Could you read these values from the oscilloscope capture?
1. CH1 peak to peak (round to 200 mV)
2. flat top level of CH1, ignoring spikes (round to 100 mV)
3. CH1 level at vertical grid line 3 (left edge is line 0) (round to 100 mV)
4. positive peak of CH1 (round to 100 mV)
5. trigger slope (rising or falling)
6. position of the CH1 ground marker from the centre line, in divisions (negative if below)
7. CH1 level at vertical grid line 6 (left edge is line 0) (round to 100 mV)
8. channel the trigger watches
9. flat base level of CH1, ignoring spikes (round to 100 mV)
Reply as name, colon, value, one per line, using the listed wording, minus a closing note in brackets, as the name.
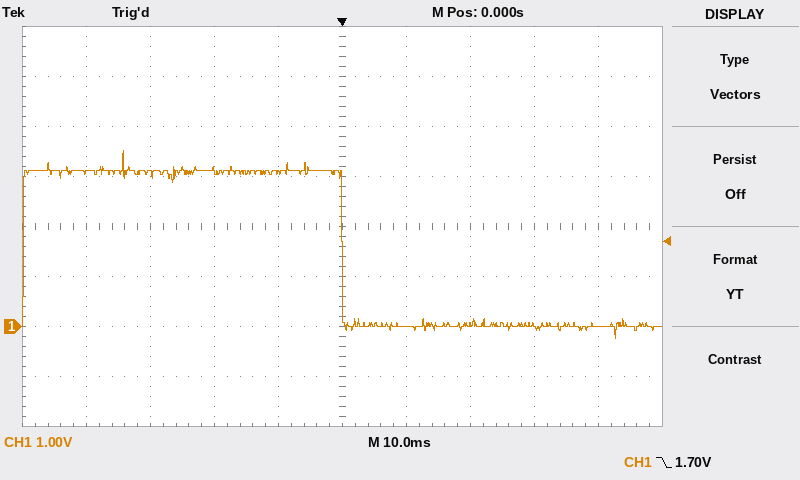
CH1 peak to peak: 3.8 V
flat top level of CH1, ignoring spikes: 3.1 V
CH1 level at vertical grid line 3 (left edge is line 0): 3.1 V
positive peak of CH1: 3.5 V
trigger slope: falling
position of the CH1 ground marker from the centre line, in divisions: -2.0 div
CH1 level at vertical grid line 6 (left edge is line 0): 0.0 V
channel the trigger watches: CH1
flat base level of CH1, ignoring spikes: 0.0 V
